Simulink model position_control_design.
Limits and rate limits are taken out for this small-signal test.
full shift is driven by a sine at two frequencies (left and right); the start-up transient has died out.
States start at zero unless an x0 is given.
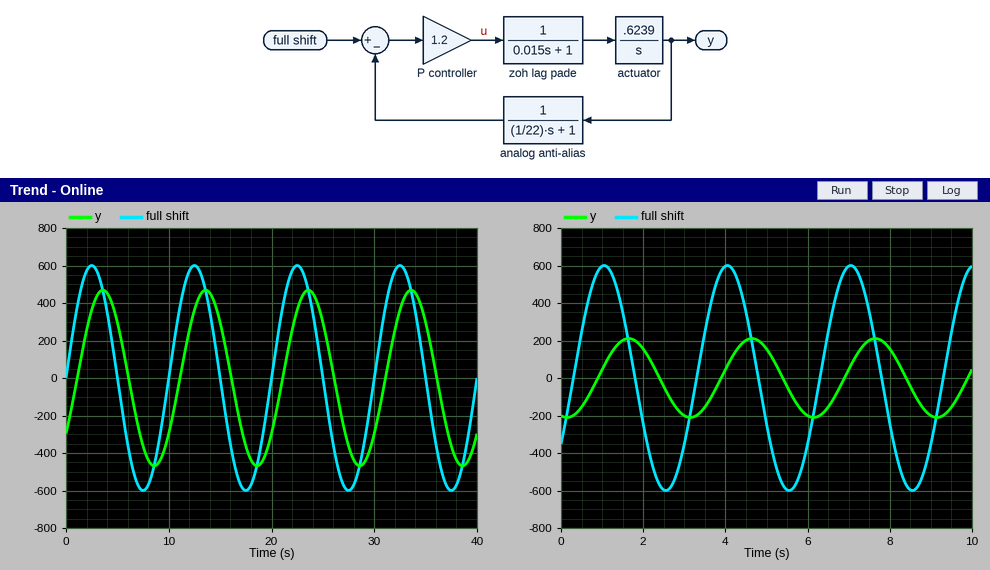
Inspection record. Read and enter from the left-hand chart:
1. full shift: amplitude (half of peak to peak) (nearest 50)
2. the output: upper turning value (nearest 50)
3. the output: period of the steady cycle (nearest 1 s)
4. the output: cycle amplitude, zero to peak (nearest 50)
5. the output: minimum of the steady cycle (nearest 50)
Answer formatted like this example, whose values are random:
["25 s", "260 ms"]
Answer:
["600", "450", "10 s", "450", "-450"]
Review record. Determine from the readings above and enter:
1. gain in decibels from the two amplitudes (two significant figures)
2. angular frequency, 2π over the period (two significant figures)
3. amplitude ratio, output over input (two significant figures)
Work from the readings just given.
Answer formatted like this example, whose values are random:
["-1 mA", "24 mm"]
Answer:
["-2.5 dB", "0.63 rad/s", "0.75"]
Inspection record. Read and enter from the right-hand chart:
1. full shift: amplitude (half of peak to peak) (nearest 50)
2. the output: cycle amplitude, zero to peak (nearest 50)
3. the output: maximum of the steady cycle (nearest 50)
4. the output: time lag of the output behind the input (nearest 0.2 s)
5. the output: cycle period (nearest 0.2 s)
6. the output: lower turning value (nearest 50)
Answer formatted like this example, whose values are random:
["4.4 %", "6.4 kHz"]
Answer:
["600", "200", "200", "0.6 s", "3.0 s", "-200"]
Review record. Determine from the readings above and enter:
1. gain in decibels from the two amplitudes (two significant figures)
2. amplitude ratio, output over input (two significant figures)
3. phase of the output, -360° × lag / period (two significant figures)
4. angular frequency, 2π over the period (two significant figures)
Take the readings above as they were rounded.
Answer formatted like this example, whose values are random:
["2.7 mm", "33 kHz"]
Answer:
["-9.5 dB", "0.33", "-72°", "2.1 rad/s"]
